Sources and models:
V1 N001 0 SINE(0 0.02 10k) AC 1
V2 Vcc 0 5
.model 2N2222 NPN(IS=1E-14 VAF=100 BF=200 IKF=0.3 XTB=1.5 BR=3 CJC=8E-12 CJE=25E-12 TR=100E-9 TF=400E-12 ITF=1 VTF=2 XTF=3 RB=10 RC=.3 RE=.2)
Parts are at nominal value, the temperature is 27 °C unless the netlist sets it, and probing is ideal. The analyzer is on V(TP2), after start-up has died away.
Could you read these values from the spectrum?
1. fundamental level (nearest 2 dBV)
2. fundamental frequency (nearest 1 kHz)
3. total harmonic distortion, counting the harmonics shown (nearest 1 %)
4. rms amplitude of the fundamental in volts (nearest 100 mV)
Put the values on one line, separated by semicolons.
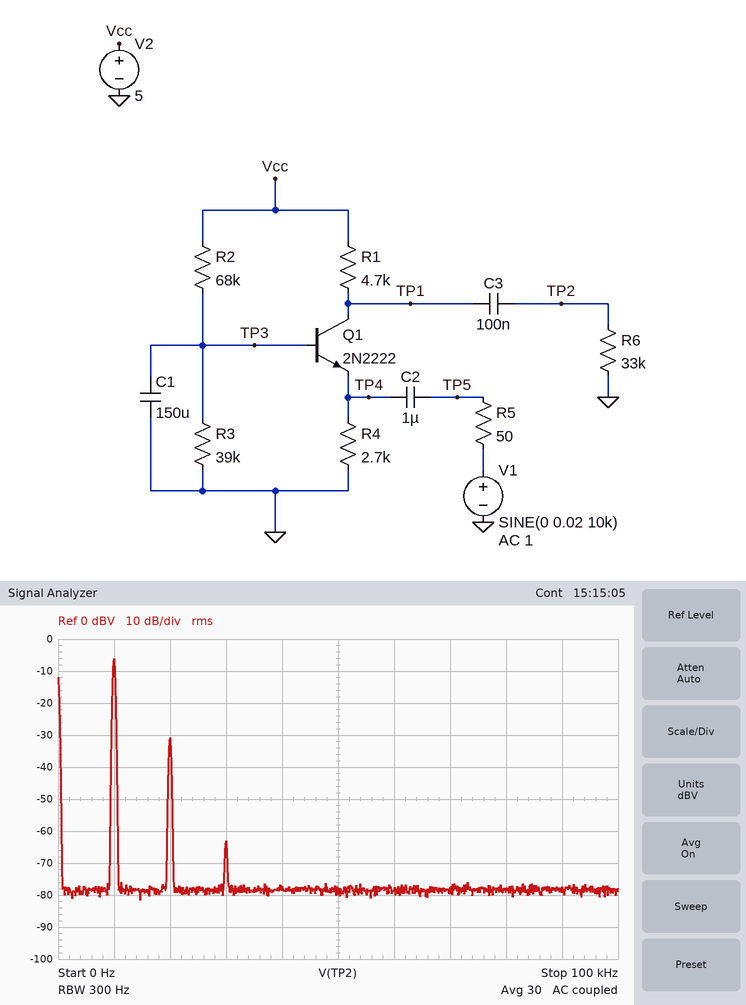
-6 dBV; 10 kHz; 6 %; 500 mV
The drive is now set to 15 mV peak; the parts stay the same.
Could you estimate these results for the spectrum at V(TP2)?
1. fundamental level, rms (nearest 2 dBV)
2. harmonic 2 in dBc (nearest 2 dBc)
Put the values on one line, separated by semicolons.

-8 dBV; -28 dBc
